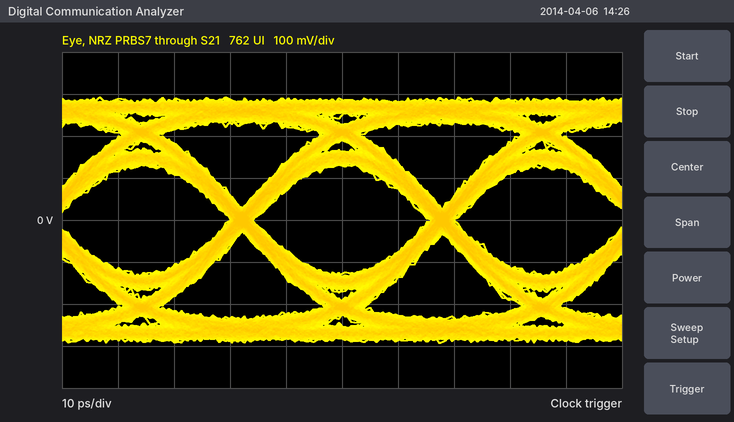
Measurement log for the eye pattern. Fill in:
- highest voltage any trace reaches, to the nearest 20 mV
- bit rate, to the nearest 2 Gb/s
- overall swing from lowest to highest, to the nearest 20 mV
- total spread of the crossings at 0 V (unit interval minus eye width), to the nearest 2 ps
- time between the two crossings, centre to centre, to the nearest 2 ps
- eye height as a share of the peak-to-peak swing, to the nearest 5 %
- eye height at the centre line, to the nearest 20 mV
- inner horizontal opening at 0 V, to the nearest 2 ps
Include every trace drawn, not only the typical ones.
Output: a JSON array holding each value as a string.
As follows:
["300 mV", "28 Gb/s", "580 mV", "4 ps", "36 ps", "45 %", "260 mV", "32 ps"]
